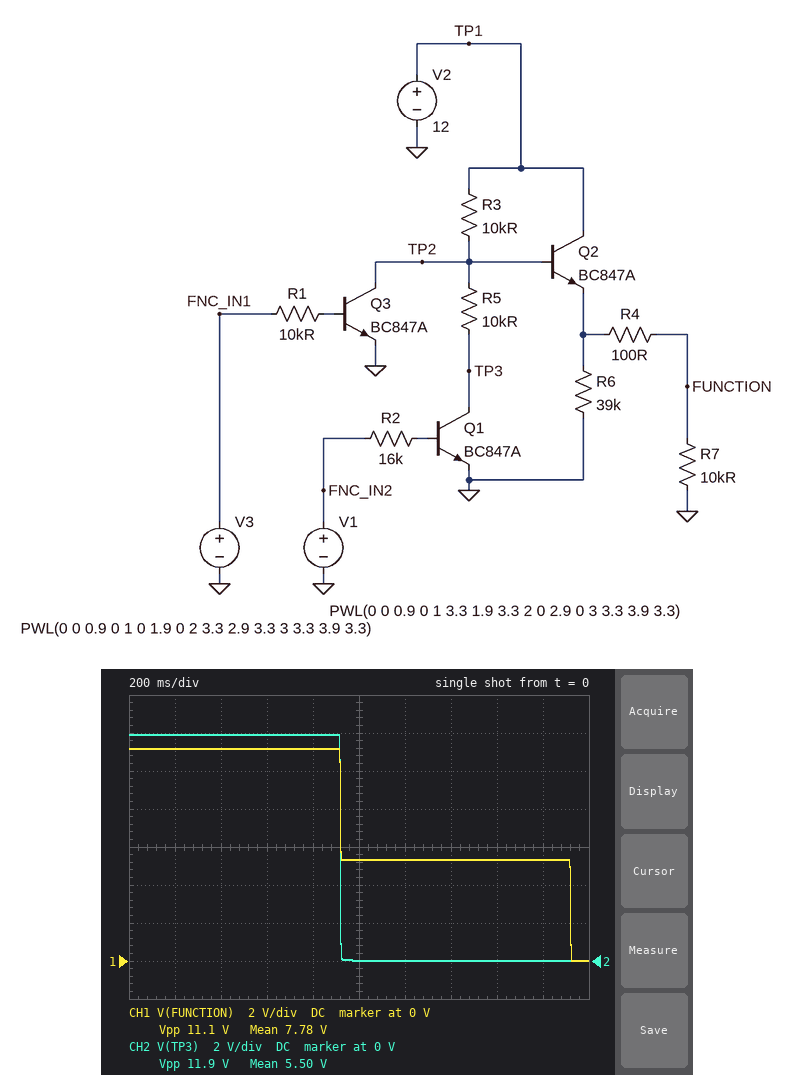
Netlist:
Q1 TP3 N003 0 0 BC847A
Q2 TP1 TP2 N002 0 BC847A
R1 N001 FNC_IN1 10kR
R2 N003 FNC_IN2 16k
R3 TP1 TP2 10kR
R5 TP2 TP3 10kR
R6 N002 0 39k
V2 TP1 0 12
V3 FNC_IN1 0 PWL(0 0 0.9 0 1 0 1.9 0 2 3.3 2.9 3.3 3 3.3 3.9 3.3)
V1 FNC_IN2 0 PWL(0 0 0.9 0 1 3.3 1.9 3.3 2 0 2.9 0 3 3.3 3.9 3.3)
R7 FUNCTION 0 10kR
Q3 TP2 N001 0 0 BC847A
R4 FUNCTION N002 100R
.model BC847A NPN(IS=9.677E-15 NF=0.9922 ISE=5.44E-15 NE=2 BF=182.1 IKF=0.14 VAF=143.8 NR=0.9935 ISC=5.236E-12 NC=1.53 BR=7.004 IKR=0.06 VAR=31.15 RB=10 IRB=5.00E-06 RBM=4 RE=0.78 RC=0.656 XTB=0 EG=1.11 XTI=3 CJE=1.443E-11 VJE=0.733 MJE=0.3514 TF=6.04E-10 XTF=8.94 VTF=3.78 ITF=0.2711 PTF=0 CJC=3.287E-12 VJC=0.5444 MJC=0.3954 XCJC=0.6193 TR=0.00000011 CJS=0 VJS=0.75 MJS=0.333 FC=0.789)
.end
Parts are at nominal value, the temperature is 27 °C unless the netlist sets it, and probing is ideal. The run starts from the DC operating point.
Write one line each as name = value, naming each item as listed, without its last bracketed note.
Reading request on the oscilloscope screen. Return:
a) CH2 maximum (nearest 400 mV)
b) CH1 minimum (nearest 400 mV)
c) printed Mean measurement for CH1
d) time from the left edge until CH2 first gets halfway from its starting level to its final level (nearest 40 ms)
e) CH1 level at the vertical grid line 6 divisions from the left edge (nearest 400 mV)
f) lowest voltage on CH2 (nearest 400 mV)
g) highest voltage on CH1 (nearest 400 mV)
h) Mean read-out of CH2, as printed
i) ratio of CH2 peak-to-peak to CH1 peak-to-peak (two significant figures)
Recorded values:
CH2 maximum = 12.0 V
CH1 minimum = 0 V
printed Mean measurement for CH1 = 7.78 V
time from the left edge until CH2 first gets halfway from its starting level to its final level = 920 ms
CH1 level at the vertical grid line 6 divisions from the left edge = 5.2 V
lowest voltage on CH2 = 0 V
highest voltage on CH1 = 11.2 V
Mean read-out of CH2, as printed = 5.50 V
ratio of CH2 peak-to-peak to CH1 peak-to-peak = 1.1
